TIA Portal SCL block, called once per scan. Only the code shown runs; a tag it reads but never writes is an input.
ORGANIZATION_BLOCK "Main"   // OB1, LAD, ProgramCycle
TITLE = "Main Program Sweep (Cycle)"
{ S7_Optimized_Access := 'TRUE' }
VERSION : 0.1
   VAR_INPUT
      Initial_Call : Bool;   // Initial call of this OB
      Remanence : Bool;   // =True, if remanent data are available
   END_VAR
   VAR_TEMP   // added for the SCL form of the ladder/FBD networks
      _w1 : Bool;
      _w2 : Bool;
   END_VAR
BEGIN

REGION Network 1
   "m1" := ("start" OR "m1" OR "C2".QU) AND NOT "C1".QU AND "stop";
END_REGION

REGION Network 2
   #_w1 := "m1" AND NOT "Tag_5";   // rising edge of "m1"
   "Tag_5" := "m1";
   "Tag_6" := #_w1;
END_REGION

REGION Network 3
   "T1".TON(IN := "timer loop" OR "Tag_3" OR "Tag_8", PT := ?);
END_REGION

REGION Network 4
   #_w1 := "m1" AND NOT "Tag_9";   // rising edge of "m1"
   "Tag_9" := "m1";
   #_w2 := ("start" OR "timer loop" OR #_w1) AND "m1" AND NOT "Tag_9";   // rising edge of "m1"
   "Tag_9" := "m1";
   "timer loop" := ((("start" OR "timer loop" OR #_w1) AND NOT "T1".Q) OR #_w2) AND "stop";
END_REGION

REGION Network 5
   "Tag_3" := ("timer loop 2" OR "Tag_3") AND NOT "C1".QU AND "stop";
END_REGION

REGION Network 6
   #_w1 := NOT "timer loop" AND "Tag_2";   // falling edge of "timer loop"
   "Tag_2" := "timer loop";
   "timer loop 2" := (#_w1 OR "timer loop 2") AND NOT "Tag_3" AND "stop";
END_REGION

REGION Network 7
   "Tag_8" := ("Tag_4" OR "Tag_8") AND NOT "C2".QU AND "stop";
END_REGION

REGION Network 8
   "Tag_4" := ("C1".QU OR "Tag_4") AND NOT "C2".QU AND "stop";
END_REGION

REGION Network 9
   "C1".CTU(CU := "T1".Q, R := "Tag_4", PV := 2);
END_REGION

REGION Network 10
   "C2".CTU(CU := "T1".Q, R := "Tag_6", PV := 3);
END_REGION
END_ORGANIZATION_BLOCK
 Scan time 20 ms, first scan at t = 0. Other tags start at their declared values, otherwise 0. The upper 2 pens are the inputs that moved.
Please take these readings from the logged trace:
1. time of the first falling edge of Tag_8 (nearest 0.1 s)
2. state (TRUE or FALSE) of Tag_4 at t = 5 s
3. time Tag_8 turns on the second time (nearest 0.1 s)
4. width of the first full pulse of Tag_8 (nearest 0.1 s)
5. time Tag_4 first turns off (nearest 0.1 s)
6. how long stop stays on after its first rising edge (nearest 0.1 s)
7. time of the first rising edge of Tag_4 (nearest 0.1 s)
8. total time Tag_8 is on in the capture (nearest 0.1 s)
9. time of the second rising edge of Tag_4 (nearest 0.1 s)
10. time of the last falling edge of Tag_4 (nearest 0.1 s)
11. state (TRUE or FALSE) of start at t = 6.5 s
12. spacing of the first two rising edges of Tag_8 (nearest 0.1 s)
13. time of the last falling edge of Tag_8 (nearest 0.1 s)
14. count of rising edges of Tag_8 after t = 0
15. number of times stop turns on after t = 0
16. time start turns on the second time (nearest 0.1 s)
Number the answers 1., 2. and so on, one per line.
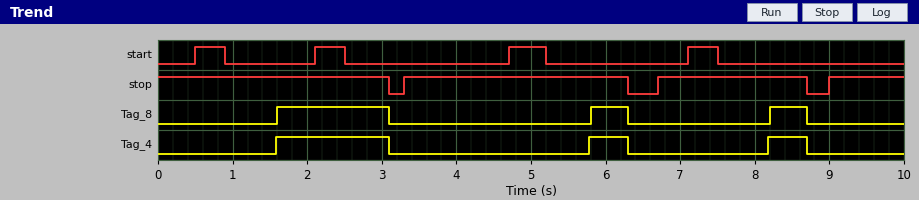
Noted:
1. 3.1 s
2. FALSE
3. 5.8 s
4. 1.5 s
5. 3.1 s
6. 3.0 s
7. 1.6 s
8. 2.5 s
9. 5.8 s
10. 8.7 s
11. FALSE
12. 4.2 s
13. 8.7 s
14. 3
15. 3
16. 2.1 s
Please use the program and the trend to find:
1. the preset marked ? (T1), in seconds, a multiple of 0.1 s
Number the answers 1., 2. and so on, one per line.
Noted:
1. 0.5 s
